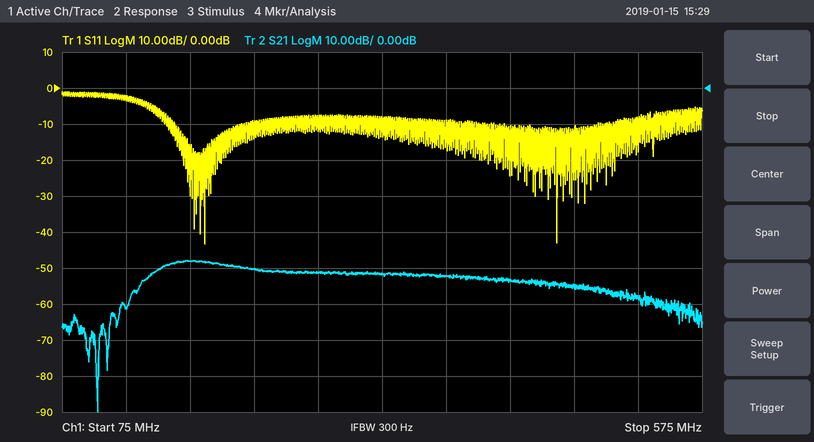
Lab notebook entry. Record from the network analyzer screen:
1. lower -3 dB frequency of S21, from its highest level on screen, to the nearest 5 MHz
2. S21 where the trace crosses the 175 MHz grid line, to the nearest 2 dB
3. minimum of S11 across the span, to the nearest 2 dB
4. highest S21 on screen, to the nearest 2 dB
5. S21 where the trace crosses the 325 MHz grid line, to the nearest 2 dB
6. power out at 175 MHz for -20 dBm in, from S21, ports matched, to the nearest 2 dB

150 MHz
-48 dB
-44 dB
-48 dB
-52 dB
-68 dBm
